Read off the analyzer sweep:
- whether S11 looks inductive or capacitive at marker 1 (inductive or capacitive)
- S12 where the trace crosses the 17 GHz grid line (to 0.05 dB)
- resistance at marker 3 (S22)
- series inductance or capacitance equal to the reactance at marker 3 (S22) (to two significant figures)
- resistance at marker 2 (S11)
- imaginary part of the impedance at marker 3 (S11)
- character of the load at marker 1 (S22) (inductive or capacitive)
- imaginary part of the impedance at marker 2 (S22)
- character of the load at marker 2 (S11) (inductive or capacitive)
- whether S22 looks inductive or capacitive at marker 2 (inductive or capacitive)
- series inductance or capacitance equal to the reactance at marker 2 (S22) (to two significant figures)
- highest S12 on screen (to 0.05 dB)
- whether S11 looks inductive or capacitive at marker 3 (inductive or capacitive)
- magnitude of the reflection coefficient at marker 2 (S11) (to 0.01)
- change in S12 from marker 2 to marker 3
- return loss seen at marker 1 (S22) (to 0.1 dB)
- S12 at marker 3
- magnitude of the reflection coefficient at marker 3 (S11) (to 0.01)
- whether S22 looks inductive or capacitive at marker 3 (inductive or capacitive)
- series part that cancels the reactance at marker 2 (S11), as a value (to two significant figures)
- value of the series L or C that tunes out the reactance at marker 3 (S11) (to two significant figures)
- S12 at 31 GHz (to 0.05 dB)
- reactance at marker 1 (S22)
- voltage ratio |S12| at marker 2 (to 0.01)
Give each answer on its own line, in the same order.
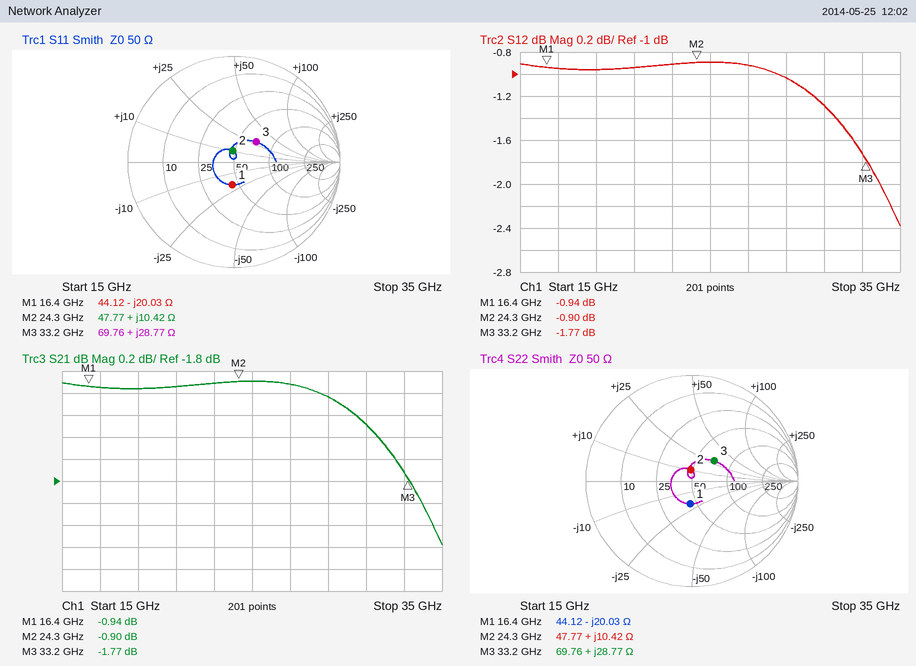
capacitive
-0.95 dB
69.76 Ω
140 pH
47.77 Ω
+28.77 Ω
capacitive
+10.42 Ω
inductive
inductive
68 pH
-0.90 dB
inductive
0.11
-0.87 dB
13.3 dB
-1.77 dB
0.28
inductive
630 fF
170 fF
-1.30 dB
-20.03 Ω
0.90
